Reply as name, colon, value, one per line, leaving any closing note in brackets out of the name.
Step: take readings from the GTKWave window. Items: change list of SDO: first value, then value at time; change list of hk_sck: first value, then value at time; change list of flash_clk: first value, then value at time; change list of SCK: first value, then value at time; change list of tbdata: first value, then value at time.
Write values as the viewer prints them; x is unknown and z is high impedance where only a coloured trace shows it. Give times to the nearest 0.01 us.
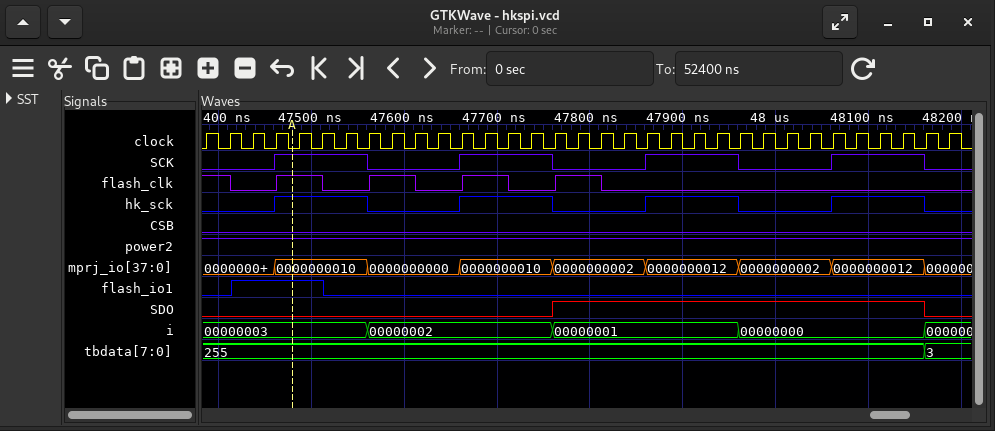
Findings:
change list of SDO: first value, then value at time: 0, 1 at 47.76 us, 0 at 48.16 us
change list of hk_sck: first value, then value at time: 0, 1 at 47.46 us, 0 at 47.56 us, 1 at 47.66 us, 0 at 47.76 us, 1 at 47.86 us, 0 at 47.96 us, 1 at 48.06 us, 0 at 48.16 us
change list of flash_clk: first value, then value at time: 1, 0 at 47.41 us, 1 at 47.46 us, 0 at 47.51 us, 1 at 47.56 us, 0 at 47.61 us, 1 at 47.66 us, 0 at 47.71 us, 1 at 47.76 us, 0 at 47.81 us
change list of SCK: first value, then value at time: 0, 1 at 47.46 us, 0 at 47.56 us, 1 at 47.66 us, 0 at 47.76 us, 1 at 47.86 us, 0 at 47.96 us, 1 at 48.06 us, 0 at 48.16 us
change list of tbdata: first value, then value at time: 255, 3 at 48.16 us
